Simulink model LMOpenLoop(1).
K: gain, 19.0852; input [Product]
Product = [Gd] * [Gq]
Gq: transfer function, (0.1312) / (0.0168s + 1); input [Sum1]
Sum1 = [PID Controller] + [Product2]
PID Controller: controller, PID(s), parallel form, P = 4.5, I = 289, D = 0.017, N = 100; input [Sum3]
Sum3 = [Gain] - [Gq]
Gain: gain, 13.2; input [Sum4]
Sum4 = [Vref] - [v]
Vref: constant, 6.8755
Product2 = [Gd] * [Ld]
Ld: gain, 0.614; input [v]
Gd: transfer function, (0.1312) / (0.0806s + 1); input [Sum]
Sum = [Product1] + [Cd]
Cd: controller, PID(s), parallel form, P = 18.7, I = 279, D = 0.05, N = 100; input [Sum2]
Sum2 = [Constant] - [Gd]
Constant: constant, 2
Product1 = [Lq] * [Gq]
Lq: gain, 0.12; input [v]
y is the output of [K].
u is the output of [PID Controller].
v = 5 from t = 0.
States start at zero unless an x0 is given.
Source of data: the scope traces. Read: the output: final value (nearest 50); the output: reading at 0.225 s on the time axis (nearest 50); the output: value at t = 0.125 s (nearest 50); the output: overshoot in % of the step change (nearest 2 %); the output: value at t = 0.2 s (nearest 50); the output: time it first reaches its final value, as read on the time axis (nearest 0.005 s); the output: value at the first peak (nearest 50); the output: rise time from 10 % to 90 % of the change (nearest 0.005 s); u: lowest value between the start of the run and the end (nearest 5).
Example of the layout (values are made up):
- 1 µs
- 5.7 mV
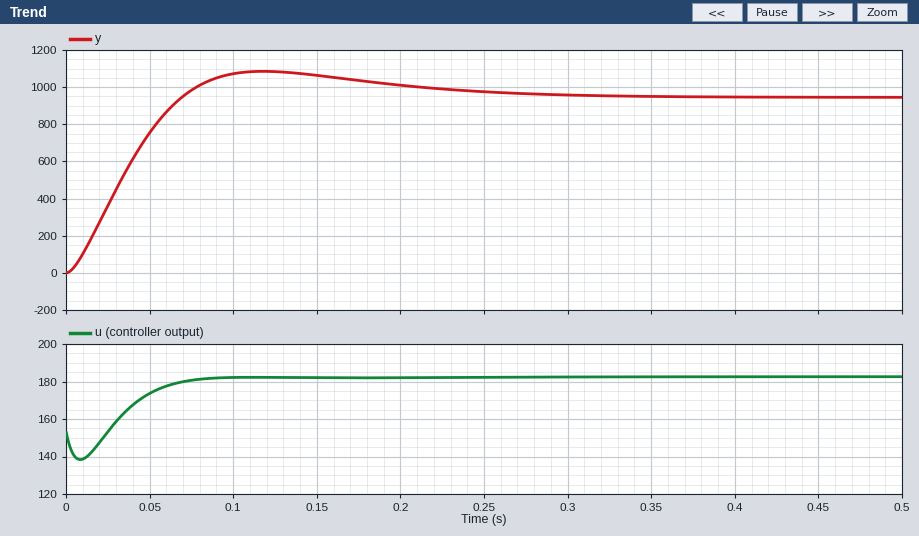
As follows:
- 950
- 1000
- 1100
- 14 %
- 1000
- 0.070 s
- 1100
- 0.050 s
- 140
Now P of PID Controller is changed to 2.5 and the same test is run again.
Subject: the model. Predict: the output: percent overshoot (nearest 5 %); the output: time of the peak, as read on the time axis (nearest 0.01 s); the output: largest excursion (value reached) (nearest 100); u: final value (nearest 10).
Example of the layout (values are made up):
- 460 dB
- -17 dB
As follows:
- 20 %
- 0.11 s
- 1100
- 180
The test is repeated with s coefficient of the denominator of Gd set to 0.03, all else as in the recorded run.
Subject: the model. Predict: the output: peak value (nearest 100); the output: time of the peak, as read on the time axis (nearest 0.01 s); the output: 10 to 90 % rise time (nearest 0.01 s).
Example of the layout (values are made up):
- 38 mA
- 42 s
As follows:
- 1000
- 0.11 s
- 0.05 s
